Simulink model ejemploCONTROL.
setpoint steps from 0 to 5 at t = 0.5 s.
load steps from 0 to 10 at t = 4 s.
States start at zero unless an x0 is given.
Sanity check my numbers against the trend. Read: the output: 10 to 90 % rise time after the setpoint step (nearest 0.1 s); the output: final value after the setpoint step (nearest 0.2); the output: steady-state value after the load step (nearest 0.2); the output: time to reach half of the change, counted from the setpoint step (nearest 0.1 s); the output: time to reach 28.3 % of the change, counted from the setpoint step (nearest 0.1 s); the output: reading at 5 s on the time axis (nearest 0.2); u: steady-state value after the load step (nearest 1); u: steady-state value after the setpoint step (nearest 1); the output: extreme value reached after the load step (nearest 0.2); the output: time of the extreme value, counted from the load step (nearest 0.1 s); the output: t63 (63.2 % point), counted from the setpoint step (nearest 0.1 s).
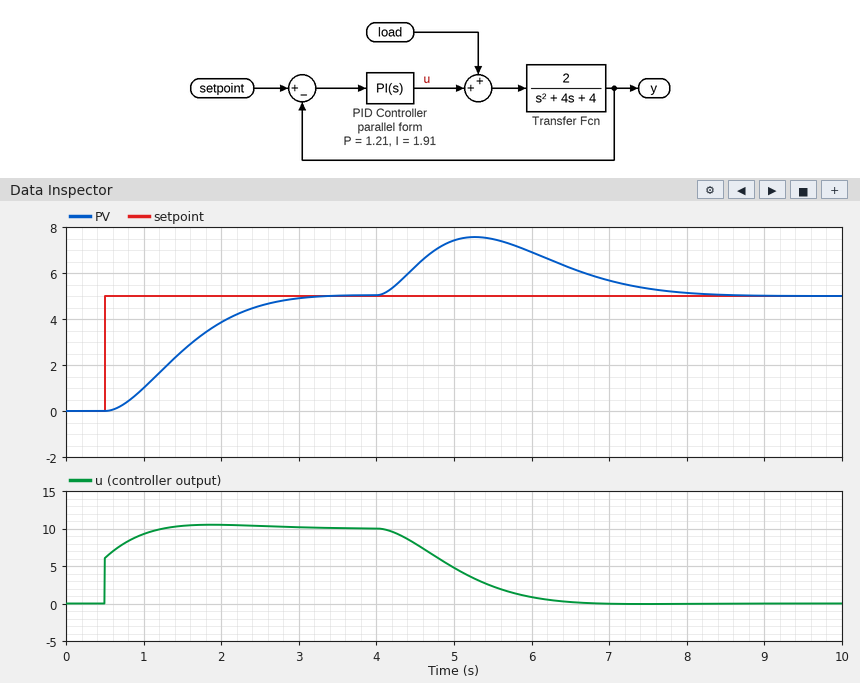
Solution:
1.6 s
5.0
5.0
1.0 s
0.6 s
7.4
0
10
7.6
1.3 s
1.2 s
